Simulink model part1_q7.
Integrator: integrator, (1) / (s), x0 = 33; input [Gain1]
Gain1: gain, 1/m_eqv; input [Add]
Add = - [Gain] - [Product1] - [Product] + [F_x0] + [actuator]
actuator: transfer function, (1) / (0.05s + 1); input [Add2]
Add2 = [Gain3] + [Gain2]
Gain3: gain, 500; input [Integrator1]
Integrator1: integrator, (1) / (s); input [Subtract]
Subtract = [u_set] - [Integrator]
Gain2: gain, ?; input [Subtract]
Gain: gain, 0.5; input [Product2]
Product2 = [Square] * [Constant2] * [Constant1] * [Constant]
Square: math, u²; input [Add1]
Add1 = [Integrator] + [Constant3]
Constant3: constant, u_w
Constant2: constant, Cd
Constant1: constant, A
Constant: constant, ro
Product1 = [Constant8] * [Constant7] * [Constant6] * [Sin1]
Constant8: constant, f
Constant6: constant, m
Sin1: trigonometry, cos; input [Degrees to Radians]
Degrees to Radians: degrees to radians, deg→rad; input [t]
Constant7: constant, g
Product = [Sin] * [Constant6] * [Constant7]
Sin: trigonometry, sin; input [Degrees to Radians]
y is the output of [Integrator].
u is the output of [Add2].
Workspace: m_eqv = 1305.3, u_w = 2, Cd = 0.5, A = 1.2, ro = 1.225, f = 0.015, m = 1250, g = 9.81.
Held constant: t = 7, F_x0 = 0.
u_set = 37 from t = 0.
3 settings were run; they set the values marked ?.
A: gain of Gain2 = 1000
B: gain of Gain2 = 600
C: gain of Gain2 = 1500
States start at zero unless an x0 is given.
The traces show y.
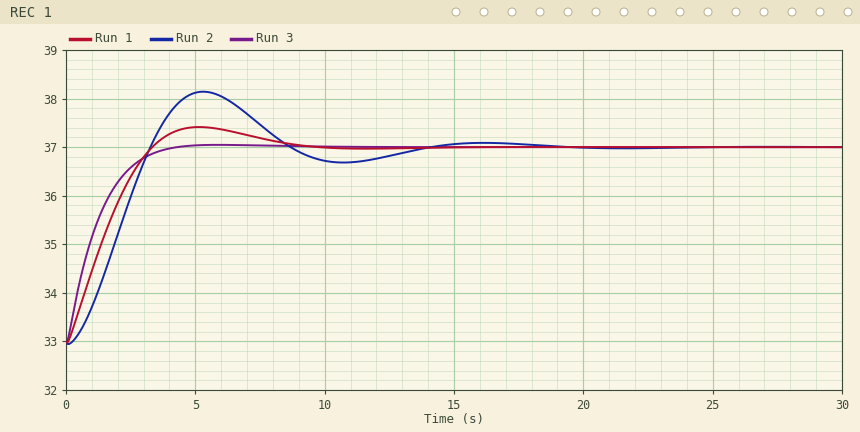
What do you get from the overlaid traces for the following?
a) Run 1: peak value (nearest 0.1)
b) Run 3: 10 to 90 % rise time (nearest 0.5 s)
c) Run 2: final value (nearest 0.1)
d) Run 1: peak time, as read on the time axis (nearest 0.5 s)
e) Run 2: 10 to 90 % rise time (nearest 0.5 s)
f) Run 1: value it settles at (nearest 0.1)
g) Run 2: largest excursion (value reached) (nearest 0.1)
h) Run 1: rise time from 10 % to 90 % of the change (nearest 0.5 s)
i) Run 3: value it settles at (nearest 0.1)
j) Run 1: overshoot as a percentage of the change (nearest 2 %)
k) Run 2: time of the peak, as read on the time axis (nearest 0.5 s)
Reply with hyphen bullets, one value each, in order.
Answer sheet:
- 37.4
- 2.5 s
- 37.0
- 5.0 s
- 2.0 s
- 37.0
- 38.1
- 2.5 s
- 37.0
- 10 %
- 5.5 s
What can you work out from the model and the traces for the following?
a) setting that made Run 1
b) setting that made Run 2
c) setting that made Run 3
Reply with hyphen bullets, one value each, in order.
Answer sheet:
- A
- B
- C
